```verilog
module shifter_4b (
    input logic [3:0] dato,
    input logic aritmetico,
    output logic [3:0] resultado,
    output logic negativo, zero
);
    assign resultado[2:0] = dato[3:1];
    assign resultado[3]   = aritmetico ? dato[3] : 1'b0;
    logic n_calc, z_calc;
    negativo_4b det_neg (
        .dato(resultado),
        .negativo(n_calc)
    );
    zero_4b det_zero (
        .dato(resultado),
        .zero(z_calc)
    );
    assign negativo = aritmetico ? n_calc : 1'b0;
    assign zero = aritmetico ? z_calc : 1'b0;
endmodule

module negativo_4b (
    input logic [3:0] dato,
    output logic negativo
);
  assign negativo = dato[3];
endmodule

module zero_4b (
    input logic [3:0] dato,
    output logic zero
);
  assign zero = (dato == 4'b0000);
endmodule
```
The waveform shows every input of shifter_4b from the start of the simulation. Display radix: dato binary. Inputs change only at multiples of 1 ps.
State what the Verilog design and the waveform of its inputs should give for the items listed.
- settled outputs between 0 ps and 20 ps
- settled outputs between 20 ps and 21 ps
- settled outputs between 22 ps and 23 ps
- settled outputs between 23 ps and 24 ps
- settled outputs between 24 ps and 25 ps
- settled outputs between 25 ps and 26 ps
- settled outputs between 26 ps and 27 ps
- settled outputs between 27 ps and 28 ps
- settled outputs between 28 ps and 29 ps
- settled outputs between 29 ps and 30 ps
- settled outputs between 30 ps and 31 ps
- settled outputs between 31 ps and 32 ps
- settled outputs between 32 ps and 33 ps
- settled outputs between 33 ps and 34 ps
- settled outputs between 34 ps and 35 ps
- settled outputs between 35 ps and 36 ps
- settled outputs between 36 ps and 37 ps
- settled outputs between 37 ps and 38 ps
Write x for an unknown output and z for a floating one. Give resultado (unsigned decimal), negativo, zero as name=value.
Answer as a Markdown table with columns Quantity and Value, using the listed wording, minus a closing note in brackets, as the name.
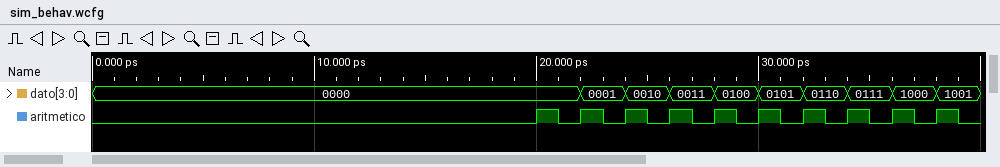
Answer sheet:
| Quantity | Value |
|---|---|
| settled outputs between 0 ps and 20 ps | resultado=0, negativo=0, zero=0 |
| settled outputs between 20 ps and 21 ps | resultado=0, negativo=0, zero=1 |
| settled outputs between 22 ps and 23 ps | resultado=0, negativo=0, zero=1 |
| settled outputs between 23 ps and 24 ps | resultado=0, negativo=0, zero=0 |
| settled outputs between 24 ps and 25 ps | resultado=1, negativo=0, zero=0 |
| settled outputs between 25 ps and 26 ps | resultado=1, negativo=0, zero=0 |
| settled outputs between 26 ps and 27 ps | resultado=1, negativo=0, zero=0 |
| settled outputs between 27 ps and 28 ps | resultado=1, negativo=0, zero=0 |
| settled outputs between 28 ps and 29 ps | resultado=2, negativo=0, zero=0 |
| settled outputs between 29 ps and 30 ps | resultado=2, negativo=0, zero=0 |
| settled outputs between 30 ps and 31 ps | resultado=2, negativo=0, zero=0 |
| settled outputs between 31 ps and 32 ps | resultado=2, negativo=0, zero=0 |
| settled outputs between 32 ps and 33 ps | resultado=3, negativo=0, zero=0 |
| settled outputs between 33 ps and 34 ps | resultado=3, negativo=0, zero=0 |
| settled outputs between 34 ps and 35 ps | resultado=3, negativo=0, zero=0 |
| settled outputs between 35 ps and 36 ps | resultado=3, negativo=0, zero=0 |
| settled outputs between 36 ps and 37 ps | resultado=12, negativo=1, zero=0 |
| settled outputs between 37 ps and 38 ps | resultado=4, negativo=0, zero=0 |
